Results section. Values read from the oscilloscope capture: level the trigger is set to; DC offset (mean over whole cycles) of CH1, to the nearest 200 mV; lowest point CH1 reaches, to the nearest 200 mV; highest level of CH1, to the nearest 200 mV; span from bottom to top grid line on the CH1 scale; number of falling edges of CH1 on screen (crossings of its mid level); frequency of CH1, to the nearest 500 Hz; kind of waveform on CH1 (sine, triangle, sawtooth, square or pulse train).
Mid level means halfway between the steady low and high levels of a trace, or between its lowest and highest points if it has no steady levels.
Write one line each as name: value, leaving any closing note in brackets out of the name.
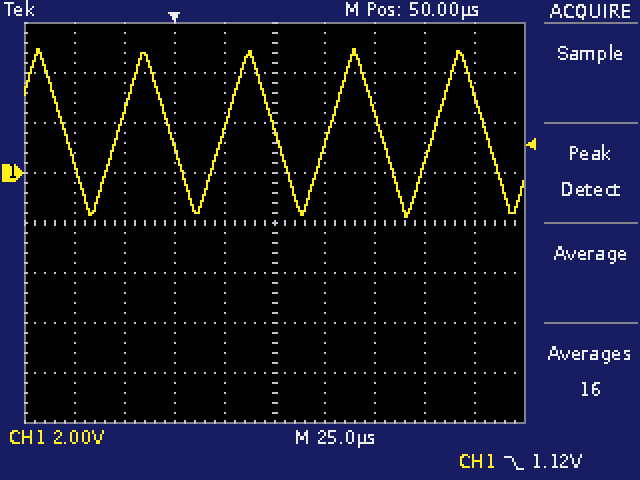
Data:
level the trigger is set to: 1.12 V
DC offset (mean over whole cycles) of CH1, to the nearest 200 mV: 1.6 V
lowest point CH1 reaches, to the nearest 200 mV: -1.8 V
highest level of CH1, to the nearest 200 mV: 5.0 V
span from bottom to top grid line on the CH1 scale: 16 V
number of falling edges of CH1 on screen: 5
frequency of CH1, to the nearest 500 Hz: 19.0 kHz
kind of waveform on CH1: triangle
